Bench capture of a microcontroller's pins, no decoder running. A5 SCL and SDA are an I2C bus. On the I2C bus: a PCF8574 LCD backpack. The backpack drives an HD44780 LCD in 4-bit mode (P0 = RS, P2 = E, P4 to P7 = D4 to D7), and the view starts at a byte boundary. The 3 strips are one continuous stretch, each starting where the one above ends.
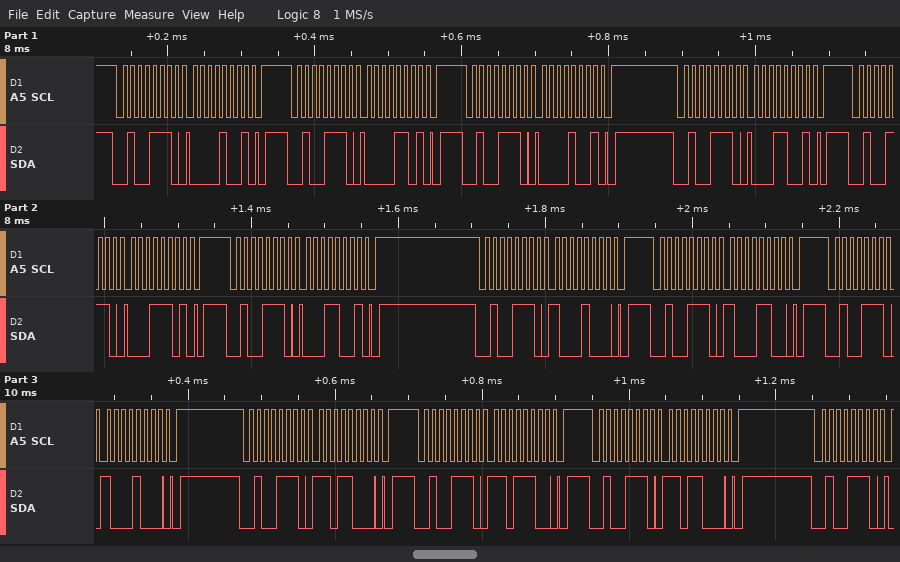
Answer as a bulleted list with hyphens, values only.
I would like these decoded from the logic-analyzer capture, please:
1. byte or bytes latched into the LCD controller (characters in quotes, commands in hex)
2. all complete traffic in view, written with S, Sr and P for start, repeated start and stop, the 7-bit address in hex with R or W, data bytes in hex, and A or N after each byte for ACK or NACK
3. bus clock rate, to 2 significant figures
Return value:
- data 0x01 0x8D
- S 27W A 09 A P S 27W A 0D A P S 27W A 09 A P S 27W A 19 A P S 27W A 1D A P S 27W A 19 A P S 27W A 88 A P S 27W A 8C A P S 27W A 88 A P S 27W A D8 A P S 27W A DC A P S 27W A D8 A P S 27W A
- 100 kHz
